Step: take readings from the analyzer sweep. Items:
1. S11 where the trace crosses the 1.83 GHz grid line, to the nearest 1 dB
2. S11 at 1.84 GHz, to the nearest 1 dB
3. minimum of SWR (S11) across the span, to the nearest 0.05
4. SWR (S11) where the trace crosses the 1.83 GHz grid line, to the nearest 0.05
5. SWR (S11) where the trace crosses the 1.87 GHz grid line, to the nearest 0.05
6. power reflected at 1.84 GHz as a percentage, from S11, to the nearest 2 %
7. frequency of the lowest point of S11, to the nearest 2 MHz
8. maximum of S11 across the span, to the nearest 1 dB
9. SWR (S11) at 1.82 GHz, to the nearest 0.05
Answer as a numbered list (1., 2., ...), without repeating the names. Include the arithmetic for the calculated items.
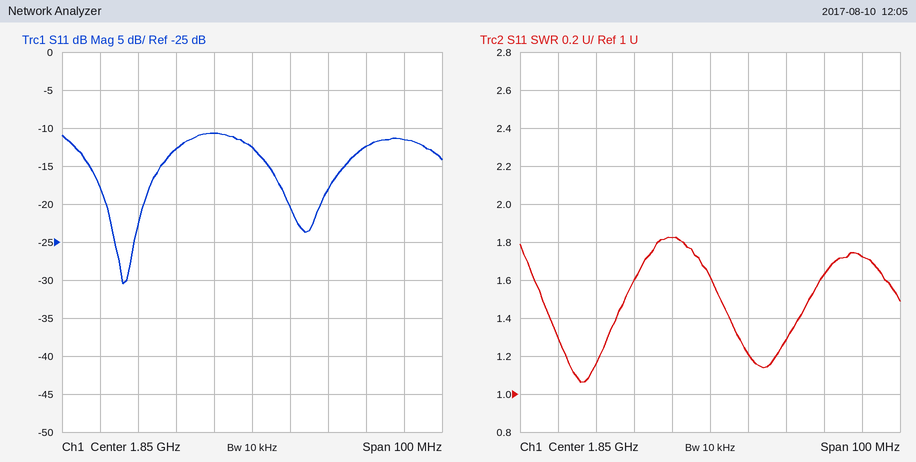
1. -13 dB
2. -11 dB
3. 1.05
4. 1.60
5. 1.30
6. 10^(-11/10) ≈ 8 %
7. 1.816 GHz
8. -11 dB
9. 1.15
